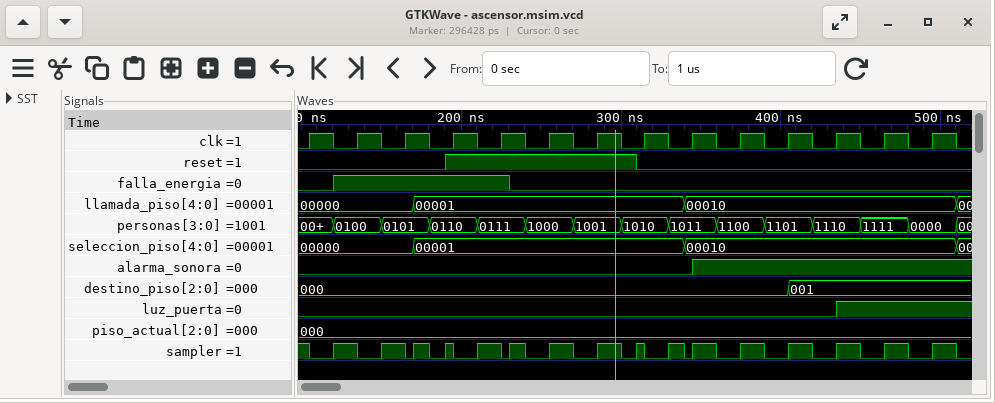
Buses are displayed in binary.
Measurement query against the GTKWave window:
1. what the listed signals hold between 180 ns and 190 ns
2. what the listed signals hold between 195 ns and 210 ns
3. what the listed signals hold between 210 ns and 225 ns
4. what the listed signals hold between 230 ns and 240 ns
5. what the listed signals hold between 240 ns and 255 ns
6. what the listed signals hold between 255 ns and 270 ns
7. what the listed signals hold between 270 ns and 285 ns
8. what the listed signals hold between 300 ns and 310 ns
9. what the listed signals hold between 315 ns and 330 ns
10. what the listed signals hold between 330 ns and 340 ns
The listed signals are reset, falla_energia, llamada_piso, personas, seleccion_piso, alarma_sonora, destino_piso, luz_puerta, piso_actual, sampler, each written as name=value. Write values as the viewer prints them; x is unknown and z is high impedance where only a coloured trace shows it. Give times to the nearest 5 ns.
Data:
reset=0, falla_energia=1, llamada_piso=00001, personas=0110, seleccion_piso=00001, alarma_sonora=0, destino_piso=000, luz_puerta=0, piso_actual=000, sampler=0
reset=1, falla_energia=1, llamada_piso=00001, personas=0110, seleccion_piso=00001, alarma_sonora=0, destino_piso=000, luz_puerta=0, piso_actual=000, sampler=0
reset=1, falla_energia=1, llamada_piso=00001, personas=0111, seleccion_piso=00001, alarma_sonora=0, destino_piso=000, luz_puerta=0, piso_actual=000, sampler=1
reset=1, falla_energia=0, llamada_piso=00001, personas=0111, seleccion_piso=00001, alarma_sonora=0, destino_piso=000, luz_puerta=0, piso_actual=000, sampler=1
reset=1, falla_energia=0, llamada_piso=00001, personas=1000, seleccion_piso=00001, alarma_sonora=0, destino_piso=000, luz_puerta=0, piso_actual=000, sampler=0
reset=1, falla_energia=0, llamada_piso=00001, personas=1000, seleccion_piso=00001, alarma_sonora=0, destino_piso=000, luz_puerta=0, piso_actual=000, sampler=1
reset=1, falla_energia=0, llamada_piso=00001, personas=1001, seleccion_piso=00001, alarma_sonora=0, destino_piso=000, luz_puerta=0, piso_actual=000, sampler=0
reset=1, falla_energia=0, llamada_piso=00001, personas=1010, seleccion_piso=00001, alarma_sonora=0, destino_piso=000, luz_puerta=0, piso_actual=000, sampler=0
reset=0, falla_energia=0, llamada_piso=00001, personas=1010, seleccion_piso=00001, alarma_sonora=0, destino_piso=000, luz_puerta=0, piso_actual=000, sampler=0
reset=0, falla_energia=0, llamada_piso=00001, personas=1011, seleccion_piso=00001, alarma_sonora=0, destino_piso=000, luz_puerta=0, piso_actual=000, sampler=1
